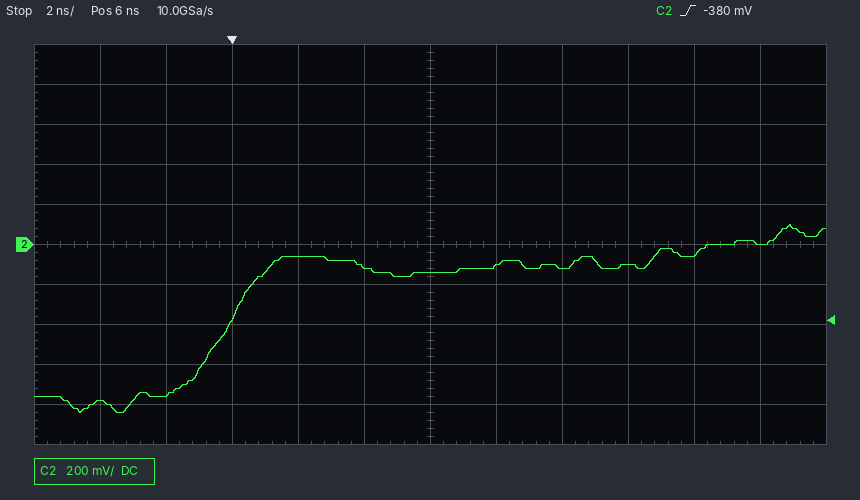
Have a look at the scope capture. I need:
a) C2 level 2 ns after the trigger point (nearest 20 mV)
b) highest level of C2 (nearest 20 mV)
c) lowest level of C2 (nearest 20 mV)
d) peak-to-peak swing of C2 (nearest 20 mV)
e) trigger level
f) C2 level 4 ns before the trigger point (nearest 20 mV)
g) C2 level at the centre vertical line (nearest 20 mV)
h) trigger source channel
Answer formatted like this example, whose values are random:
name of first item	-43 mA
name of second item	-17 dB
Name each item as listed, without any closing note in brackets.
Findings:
C2 level 2 ns after the trigger point	-60 mV
highest level of C2	100 mV
lowest level of C2	-840 mV
peak-to-peak swing of C2	940 mV
trigger level	-380 mV
C2 level 4 ns before the trigger point	-780 mV
C2 level at the centre vertical line	-140 mV
trigger source channel	C2
